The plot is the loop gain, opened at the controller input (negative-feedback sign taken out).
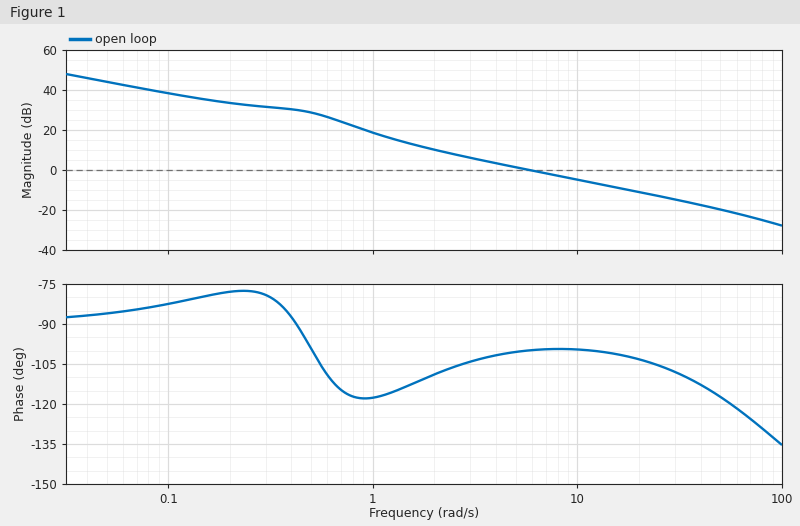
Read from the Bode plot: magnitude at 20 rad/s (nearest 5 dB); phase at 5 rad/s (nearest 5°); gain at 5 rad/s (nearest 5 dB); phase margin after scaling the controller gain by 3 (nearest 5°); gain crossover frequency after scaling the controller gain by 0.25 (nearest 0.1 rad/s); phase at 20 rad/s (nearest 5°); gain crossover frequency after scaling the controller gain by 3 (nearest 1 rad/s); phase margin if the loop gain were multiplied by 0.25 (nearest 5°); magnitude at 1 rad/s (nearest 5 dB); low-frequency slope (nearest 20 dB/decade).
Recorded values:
-10 dB
-100°
0 dB
80°
1.7 rad/s
-105°
17 rad/s
70°
20 dB
-20 dB/decade
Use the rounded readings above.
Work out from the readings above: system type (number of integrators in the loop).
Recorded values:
1
